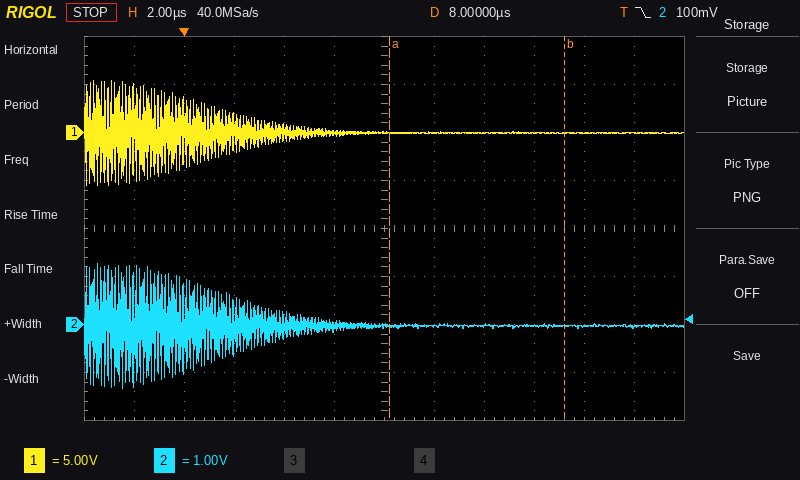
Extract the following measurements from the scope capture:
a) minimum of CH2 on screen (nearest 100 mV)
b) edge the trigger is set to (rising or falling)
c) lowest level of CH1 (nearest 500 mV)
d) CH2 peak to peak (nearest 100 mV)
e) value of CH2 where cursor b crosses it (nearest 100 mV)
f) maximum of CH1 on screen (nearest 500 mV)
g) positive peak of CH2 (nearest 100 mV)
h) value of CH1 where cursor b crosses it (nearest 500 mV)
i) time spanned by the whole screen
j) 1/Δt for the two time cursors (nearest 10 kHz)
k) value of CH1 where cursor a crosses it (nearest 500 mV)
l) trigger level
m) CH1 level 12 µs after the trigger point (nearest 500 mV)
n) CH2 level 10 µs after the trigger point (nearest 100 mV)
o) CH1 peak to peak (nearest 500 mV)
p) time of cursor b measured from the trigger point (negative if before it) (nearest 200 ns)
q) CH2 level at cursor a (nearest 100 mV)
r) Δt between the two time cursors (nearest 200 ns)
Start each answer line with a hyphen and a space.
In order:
- -1.3 V
- falling
- -5.5 V
- 2.6 V
- 0.0 V
- 5.5 V
- 1.3 V
- 0.0 V
- 24 µs
- 140 kHz
- 0.0 V
- 100 mV
- 0.0 V
- 0.0 V
- 11.0 V
- +15.2 µs
- 0.0 V
- 7.0 µs
